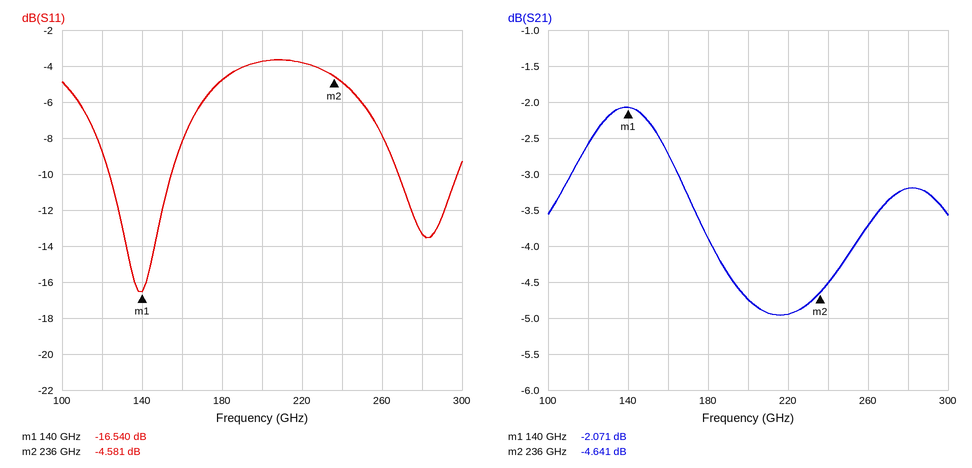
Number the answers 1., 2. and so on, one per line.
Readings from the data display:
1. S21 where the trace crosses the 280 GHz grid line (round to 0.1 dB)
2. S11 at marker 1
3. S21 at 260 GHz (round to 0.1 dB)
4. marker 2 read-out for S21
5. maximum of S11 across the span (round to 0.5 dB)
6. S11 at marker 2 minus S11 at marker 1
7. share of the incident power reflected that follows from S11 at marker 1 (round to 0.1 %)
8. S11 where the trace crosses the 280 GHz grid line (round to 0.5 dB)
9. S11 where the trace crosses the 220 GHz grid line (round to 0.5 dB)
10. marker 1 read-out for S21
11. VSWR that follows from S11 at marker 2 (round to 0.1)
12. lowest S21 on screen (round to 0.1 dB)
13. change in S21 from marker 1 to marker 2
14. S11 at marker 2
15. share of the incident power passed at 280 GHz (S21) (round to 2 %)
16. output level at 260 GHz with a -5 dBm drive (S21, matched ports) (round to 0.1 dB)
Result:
1. -3.2 dB
2. -16.540 dB
3. -3.7 dB
4. -4.641 dB
5. -3.5 dB
6. 11.959 dB
7. 2.2 %
8. -13.5 dB
9. -4.0 dB
10. -2.071 dB
11. 3.9
12. -5.0 dB
13. -2.570 dB
14. -4.581 dB
15. 48 %
16. -8.7 dBm
